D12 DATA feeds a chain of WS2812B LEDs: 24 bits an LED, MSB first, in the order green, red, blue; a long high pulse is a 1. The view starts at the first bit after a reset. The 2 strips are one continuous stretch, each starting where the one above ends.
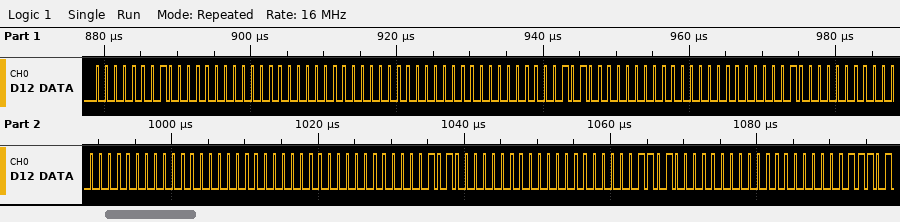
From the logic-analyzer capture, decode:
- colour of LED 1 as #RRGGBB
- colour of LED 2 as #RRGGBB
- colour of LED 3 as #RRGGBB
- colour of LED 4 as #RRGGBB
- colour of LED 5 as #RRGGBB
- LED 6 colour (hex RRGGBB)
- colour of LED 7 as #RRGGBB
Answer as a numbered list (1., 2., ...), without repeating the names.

1. #000100
2. #000000
3. #001400
4. #000800
5. #000000
6. #000500
7. #000D00
